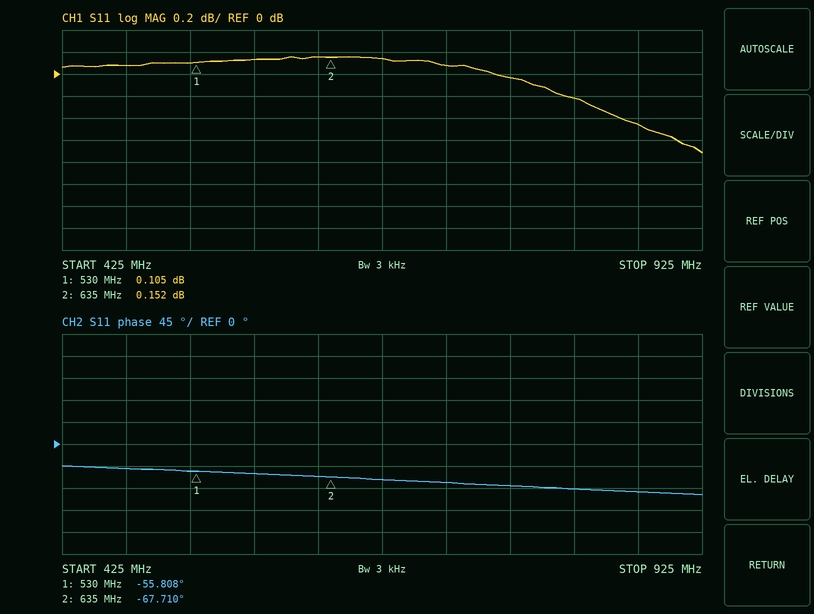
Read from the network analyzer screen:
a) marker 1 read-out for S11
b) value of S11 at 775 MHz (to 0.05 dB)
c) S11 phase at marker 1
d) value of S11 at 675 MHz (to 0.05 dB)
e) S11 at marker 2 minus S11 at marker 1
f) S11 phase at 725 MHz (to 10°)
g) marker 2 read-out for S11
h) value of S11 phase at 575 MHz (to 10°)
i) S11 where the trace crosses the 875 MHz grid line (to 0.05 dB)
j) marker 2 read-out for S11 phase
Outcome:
0.105 dB
-0.05 dB
-55.808°
0.15 dB
0.047 dB
-80°
0.152 dB
-60°
-0.45 dB
-67.710°
